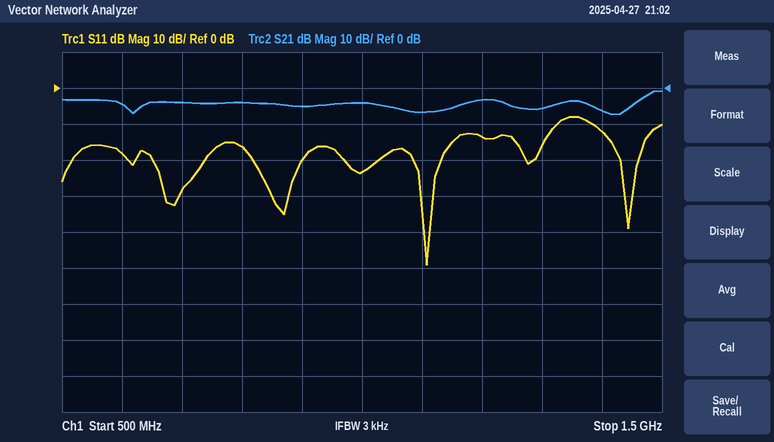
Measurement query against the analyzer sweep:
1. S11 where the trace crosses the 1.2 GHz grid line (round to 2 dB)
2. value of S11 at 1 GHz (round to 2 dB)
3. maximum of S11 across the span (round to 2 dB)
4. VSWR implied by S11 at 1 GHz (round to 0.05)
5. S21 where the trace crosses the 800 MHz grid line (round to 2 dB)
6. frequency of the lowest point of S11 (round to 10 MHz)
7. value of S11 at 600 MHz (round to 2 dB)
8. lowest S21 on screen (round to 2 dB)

-14 dB
-24 dB
-8 dB
1.15
-4 dB
1.11 GHz
-18 dB
-8 dB
